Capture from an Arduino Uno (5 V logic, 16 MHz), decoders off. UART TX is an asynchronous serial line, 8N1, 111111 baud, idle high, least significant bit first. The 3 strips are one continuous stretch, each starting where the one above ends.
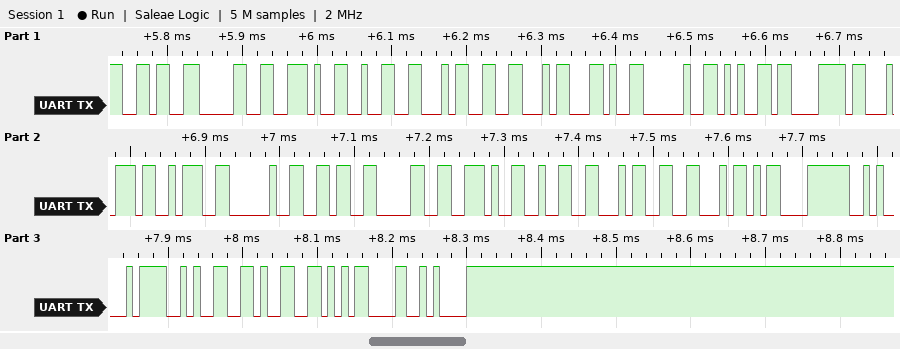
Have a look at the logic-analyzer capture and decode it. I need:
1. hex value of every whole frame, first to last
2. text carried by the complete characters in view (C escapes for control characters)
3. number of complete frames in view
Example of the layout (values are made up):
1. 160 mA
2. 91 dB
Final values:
1. 36 30 2E 32 34 46 2C 20 65 78 74 3A 20 36 30 2E 32 34 46 0D 0A 4F 66 66 0D 0A
2. "60.24F, ext: 60.24F\r\nOff\r\n"
3. 26
